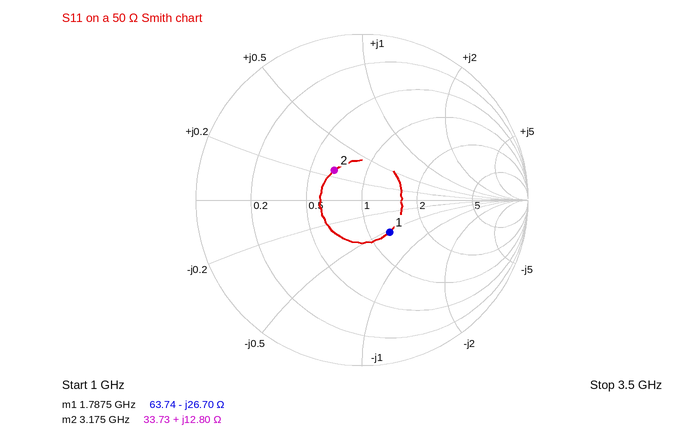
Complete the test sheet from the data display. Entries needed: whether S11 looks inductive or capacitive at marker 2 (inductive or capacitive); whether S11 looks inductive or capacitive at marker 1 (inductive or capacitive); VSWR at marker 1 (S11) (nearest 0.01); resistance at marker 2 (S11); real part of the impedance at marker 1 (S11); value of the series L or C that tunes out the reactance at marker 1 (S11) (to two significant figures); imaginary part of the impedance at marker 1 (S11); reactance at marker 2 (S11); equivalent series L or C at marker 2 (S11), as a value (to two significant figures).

inductive
capacitive
1.69
33.73 Ω
63.74 Ω
2.4 nH
-26.70 Ω
+12.80 Ω
640 pH
